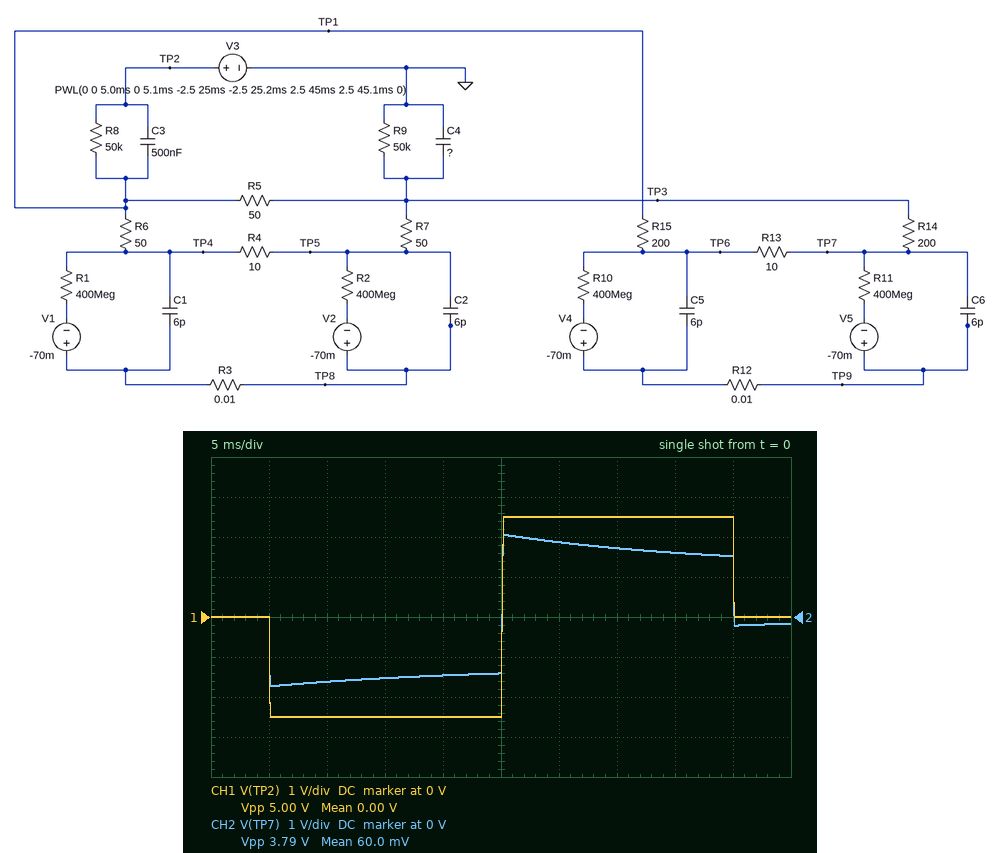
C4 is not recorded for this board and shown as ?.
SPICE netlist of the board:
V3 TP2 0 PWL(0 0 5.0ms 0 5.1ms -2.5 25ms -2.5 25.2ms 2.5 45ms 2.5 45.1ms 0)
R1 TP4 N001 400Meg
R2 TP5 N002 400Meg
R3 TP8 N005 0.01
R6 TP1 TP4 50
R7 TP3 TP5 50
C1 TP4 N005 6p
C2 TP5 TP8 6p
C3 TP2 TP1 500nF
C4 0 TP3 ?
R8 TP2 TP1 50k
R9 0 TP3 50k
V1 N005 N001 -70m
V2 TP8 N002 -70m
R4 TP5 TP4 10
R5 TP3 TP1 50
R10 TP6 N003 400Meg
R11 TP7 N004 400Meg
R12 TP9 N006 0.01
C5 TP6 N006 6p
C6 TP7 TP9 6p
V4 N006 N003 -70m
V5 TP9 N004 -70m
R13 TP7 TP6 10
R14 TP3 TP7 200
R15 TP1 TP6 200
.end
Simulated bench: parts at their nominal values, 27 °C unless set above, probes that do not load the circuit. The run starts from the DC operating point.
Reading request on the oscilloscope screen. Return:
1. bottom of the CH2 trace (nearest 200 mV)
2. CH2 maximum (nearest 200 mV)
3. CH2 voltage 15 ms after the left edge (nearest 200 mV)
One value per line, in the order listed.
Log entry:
-1.8 V
2.0 V
-1.6 V
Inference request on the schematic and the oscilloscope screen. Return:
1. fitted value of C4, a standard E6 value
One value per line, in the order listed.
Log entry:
220 nF
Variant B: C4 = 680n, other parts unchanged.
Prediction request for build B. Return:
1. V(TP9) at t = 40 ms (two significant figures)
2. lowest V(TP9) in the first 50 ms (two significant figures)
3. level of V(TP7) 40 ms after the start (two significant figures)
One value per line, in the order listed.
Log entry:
1.0 V
-1.2 V
1.1 V
